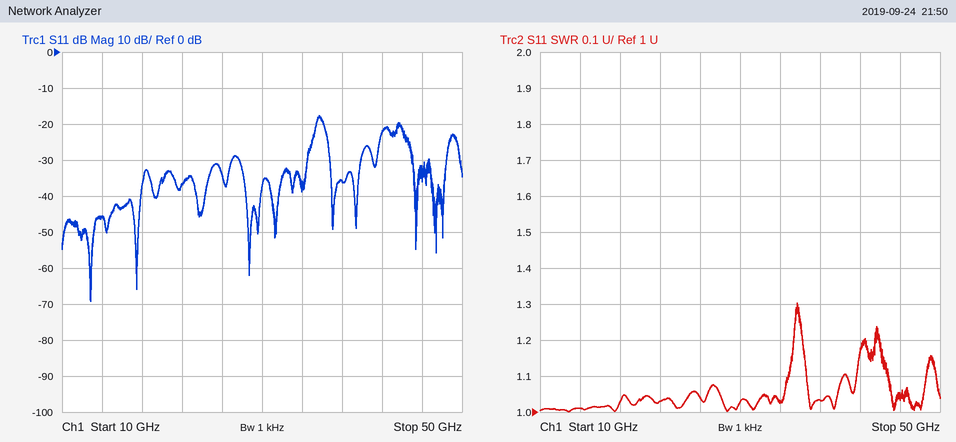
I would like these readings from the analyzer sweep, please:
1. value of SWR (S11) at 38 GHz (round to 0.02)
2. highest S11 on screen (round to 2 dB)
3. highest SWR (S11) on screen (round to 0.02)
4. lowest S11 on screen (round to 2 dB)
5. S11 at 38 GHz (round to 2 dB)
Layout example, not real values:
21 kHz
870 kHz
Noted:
1.04
-18 dB
1.30
-70 dB
-36 dB
